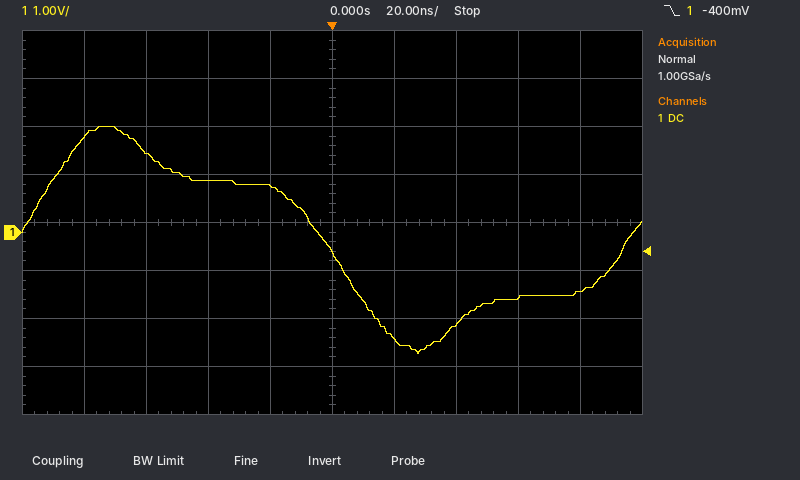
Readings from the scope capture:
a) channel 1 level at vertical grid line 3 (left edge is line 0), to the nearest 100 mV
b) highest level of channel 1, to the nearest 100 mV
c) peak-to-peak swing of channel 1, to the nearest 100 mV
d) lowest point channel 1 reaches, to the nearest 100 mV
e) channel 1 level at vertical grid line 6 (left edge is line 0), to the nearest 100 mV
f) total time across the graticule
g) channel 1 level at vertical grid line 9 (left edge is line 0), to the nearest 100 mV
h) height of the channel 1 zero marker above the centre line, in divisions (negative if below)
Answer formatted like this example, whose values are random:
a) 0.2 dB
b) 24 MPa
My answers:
a) 1.1 V
b) 2.2 V
c) 4.7 V
d) -2.5 V
e) -2.2 V
f) 200 ns
g) -1.2 V
h) -0.2 div
